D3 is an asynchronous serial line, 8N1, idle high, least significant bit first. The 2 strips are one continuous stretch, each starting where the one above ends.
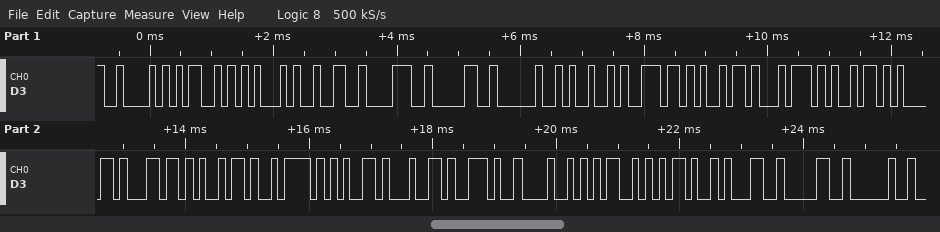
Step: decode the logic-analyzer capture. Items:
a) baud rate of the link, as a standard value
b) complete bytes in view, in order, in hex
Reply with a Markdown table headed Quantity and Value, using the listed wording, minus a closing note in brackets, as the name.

| Quantity | Value |
|---|---|
| baud rate of the link, as a standard value | 9600 baud |
| complete bytes in view, in order, in hex | 42 4D 45 32 38 30 20 49 6E 69 74 69 61 6C 69 7A 65 64 2E 48 4D 2D 31 30 20 |
